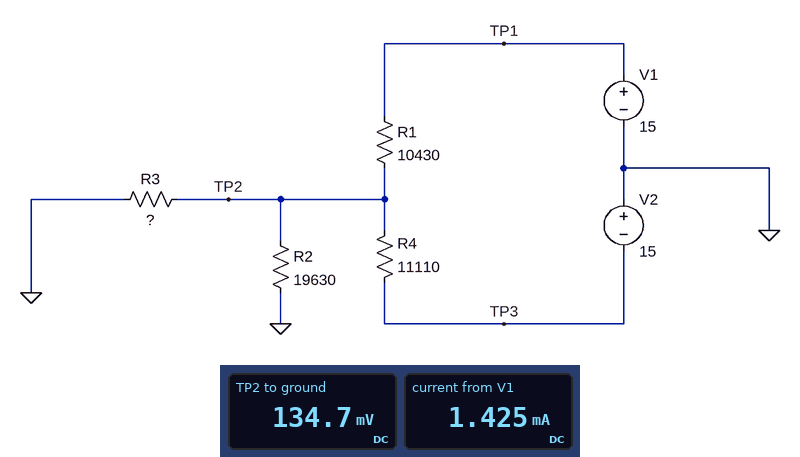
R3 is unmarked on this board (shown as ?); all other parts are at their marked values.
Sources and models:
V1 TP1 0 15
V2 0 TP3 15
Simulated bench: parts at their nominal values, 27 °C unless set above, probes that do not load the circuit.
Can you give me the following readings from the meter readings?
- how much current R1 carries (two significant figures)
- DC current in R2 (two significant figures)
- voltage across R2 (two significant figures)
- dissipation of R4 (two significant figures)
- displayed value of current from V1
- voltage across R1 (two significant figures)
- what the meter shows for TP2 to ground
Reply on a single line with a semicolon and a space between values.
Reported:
1.4 mA; 6.9 µA; 130 mV; 21 mW; 1.425 mA; 15 V; 134.7 mV
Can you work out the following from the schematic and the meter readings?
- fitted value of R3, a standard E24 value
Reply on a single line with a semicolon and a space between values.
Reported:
2.4 kΩ
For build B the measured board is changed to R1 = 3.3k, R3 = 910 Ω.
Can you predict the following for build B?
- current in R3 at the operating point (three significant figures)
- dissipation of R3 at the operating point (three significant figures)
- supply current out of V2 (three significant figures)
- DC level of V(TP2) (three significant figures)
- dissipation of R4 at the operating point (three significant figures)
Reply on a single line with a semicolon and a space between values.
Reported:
2.28 mA; 4.71 mW; 1.54 mA; 2.07 V; 26.2 mW
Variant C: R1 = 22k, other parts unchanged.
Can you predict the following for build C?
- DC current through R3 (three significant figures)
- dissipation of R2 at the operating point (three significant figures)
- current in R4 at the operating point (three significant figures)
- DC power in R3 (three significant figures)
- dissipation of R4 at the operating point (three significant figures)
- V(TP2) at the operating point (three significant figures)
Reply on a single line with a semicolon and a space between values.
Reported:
462 µA; 62.6 µW; 1.25 mA; 512 µW; 17.4 mW; -1.11 V
